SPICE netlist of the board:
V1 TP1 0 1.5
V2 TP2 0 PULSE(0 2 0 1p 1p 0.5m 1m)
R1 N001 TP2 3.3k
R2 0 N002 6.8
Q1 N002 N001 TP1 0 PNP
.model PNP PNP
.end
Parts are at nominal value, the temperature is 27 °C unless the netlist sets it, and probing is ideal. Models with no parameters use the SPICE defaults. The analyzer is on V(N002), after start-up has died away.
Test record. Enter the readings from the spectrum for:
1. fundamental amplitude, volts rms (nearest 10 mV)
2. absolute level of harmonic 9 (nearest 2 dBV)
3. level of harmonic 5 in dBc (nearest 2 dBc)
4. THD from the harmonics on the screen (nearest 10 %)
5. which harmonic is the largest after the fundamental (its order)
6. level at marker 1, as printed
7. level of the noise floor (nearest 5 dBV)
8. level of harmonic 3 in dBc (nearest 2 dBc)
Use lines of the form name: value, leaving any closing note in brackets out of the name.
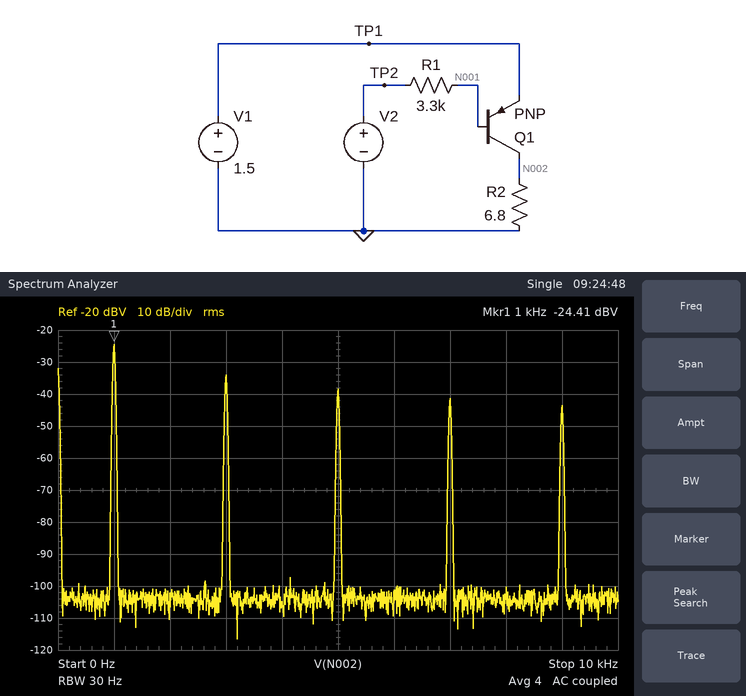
fundamental amplitude, volts rms: 60 mV
absolute level of harmonic 9: -44 dBV
level of harmonic 5 in dBc: -14 dBc
THD from the harmonics on the screen: 40 %
which harmonic is the largest after the fundamental: 3
level at marker 1, as printed: -24.41 dBV
level of the noise floor: -105 dBV
level of harmonic 3 in dBc: -10 dBc
